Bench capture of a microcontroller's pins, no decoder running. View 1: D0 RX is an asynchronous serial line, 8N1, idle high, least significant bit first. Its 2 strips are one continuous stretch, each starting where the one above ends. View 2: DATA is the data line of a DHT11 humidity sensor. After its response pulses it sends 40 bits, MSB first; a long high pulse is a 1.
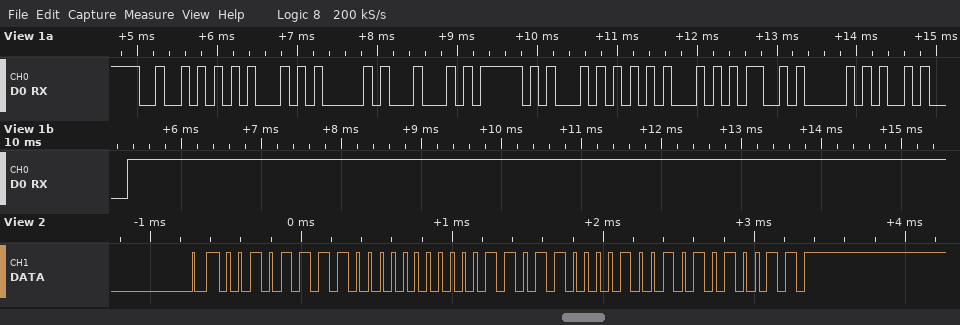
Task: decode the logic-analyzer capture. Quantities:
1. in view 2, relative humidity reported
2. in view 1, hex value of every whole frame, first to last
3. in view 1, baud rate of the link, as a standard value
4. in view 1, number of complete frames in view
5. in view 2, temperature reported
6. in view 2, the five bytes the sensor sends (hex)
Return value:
47 %
52 45 41 44 5F 54 45 4D 50 0A
9600 baud
10
27.9 °C
2F 00 1B 09 53
